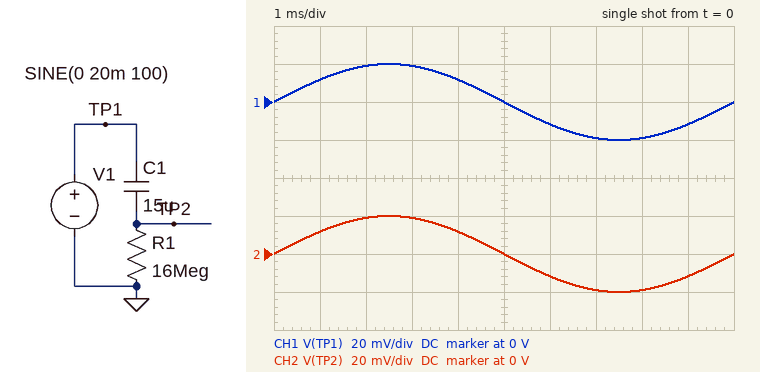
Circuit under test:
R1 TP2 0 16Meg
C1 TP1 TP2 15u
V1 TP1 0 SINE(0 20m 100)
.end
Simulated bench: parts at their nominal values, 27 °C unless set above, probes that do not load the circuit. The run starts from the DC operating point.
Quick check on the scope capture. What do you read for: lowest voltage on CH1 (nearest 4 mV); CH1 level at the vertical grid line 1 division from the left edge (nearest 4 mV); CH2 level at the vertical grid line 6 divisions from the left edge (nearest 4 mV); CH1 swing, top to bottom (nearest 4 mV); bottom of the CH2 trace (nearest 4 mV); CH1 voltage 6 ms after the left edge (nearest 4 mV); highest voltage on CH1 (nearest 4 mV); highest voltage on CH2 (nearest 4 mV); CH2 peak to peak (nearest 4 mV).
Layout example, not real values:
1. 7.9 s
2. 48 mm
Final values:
1. -20 mV
2. 12 mV
3. -12 mV
4. 40 mV
5. -20 mV
6. -12 mV
7. 20 mV
8. 20 mV
9. 40 mV
